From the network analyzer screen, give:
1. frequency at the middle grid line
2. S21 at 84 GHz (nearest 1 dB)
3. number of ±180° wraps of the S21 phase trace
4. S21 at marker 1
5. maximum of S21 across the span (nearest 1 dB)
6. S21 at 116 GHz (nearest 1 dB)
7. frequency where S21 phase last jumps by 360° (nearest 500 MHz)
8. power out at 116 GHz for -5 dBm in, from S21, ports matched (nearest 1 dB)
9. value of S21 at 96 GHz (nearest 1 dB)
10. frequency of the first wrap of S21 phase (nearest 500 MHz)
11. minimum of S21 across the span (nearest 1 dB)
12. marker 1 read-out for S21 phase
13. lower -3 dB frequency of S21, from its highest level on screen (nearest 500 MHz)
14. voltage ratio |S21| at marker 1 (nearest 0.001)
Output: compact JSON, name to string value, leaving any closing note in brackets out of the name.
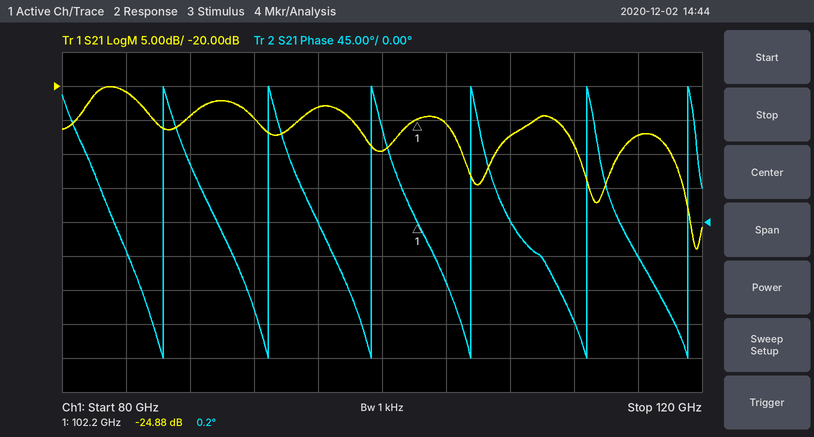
{"frequency at the middle grid line": "100 GHz", "S21 at 84 GHz": "-21 dB", "number of ±180° wraps of the S21 phase trace": "6", "S21 at marker 1": "-24.88 dB", "maximum of S21 across the span": "-20 dB", "S21 at 116 GHz": "-27 dB", "frequency where S21 phase last jumps by 360°": "119.0 GHz", "power out at 116 GHz for -5 dBm in, from S21, ports matched": "-32 dBm", "value of S21 at 96 GHz": "-23 dB", "frequency of the first wrap of S21 phase": "86.5 GHz", "minimum of S21 across the span": "-44 dB", "marker 1 read-out for S21 phase": "0.2°", "lower -3 dB frequency of S21, from its highest level on screen": "81.5 GHz", "voltage ratio |S21| at marker 1": "0.057"}
